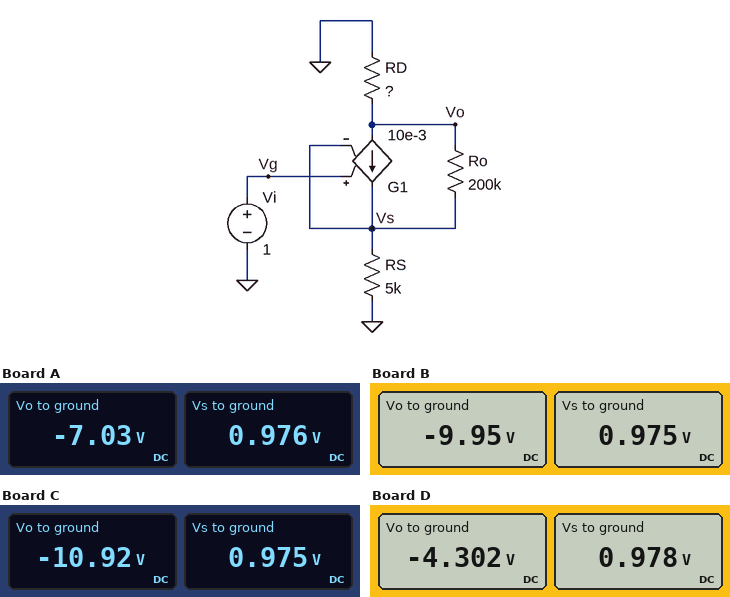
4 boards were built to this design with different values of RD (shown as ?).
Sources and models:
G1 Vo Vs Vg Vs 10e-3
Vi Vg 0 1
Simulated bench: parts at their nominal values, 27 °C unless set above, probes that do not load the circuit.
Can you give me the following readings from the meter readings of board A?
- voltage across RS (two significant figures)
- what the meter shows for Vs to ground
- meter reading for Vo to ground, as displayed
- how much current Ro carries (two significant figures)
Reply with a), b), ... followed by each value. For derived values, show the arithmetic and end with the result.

a) 976 mV = 980 mV
b) 0.976 V
c) -7.03 V
d) (976 mV - (-7.03 V)) / 200 kΩ = 40 µA
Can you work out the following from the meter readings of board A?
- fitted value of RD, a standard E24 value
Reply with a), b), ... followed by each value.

a) 36 kΩ
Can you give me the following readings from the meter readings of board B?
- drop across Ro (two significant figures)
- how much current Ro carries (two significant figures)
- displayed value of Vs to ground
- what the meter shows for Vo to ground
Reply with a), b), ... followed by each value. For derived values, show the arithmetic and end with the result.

a) 975 mV - (-9.95 V) = 11 V
b) (975 mV - (-9.95 V)) / 200 kΩ = 55 µA
c) 0.975 V
d) -9.95 V
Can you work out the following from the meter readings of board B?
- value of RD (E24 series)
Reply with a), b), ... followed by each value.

a) 51 kΩ
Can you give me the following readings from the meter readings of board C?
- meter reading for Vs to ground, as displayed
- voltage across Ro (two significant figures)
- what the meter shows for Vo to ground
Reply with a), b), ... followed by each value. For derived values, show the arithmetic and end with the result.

a) 0.975 V
b) 975 mV - (-10.92 V) = 12 V
c) -10.92 V
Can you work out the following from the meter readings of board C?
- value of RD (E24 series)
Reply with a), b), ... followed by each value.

a) 56 kΩ
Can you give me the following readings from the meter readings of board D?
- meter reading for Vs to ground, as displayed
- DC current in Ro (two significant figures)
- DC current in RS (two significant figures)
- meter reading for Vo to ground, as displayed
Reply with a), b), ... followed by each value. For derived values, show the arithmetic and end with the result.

a) 0.978 V
b) (978 mV - (-4.302 V)) / 200 kΩ = 26 µA
c) (978 mV) / 5 kΩ = 200 µA
d) -4.302 V
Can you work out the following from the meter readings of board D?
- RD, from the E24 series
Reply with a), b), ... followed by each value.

a) 22 kΩ
